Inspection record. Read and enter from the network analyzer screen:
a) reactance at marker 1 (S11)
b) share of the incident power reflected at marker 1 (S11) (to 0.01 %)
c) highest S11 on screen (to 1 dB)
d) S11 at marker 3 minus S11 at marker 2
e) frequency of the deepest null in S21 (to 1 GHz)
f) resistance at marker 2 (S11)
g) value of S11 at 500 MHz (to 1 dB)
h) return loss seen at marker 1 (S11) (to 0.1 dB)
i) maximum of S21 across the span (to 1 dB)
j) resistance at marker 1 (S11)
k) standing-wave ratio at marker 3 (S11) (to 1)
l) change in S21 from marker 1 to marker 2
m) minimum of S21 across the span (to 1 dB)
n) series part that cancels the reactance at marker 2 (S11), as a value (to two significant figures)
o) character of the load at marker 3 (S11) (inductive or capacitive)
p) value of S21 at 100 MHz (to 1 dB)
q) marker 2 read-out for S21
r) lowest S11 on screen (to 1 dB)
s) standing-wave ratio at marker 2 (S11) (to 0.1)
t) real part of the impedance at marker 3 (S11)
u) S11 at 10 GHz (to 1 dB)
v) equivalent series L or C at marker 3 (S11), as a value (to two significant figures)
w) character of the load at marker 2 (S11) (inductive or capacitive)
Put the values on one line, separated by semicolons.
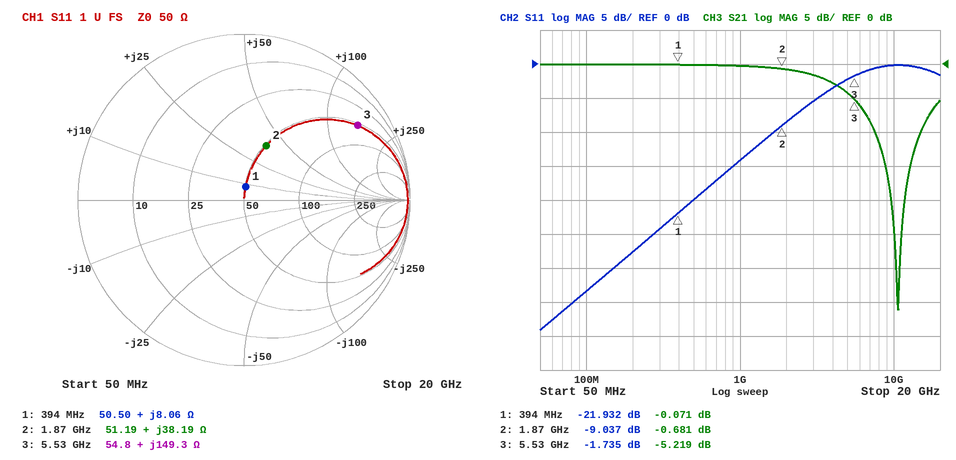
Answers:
+8.06 Ω; 0.64 %; 0 dB; 7.302 dB; 11 GHz; 51.19 Ω; -20 dB; 21.9 dB; 0 dB; 50.50 Ω; 10; -0.610 dB; -36 dB; 2.2 pF; inductive; 0 dB; -0.681 dB; -39 dB; 2.1; 54.8 Ω; 0 dB; 4.3 nH; inductive
